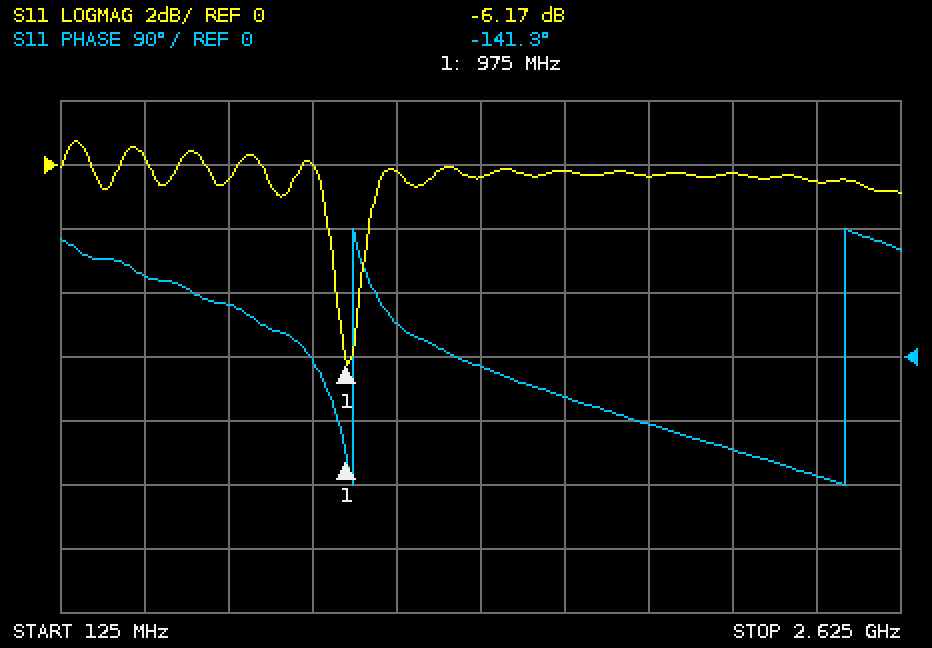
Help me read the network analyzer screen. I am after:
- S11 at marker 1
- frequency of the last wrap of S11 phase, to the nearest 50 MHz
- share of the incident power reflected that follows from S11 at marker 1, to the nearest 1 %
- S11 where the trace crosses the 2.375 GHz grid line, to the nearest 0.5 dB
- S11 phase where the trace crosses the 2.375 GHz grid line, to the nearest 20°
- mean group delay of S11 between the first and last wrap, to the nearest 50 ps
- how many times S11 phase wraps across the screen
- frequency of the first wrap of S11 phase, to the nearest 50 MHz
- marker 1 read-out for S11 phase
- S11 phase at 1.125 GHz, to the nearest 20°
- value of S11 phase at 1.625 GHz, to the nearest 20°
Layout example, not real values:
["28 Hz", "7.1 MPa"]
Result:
["-6.17 dB", "2.45 GHz", "24 %", "-0.5 dB", "-160°", "700 ps", "2", "1.00 GHz", "-141.3°", "40°", "-60°"]
